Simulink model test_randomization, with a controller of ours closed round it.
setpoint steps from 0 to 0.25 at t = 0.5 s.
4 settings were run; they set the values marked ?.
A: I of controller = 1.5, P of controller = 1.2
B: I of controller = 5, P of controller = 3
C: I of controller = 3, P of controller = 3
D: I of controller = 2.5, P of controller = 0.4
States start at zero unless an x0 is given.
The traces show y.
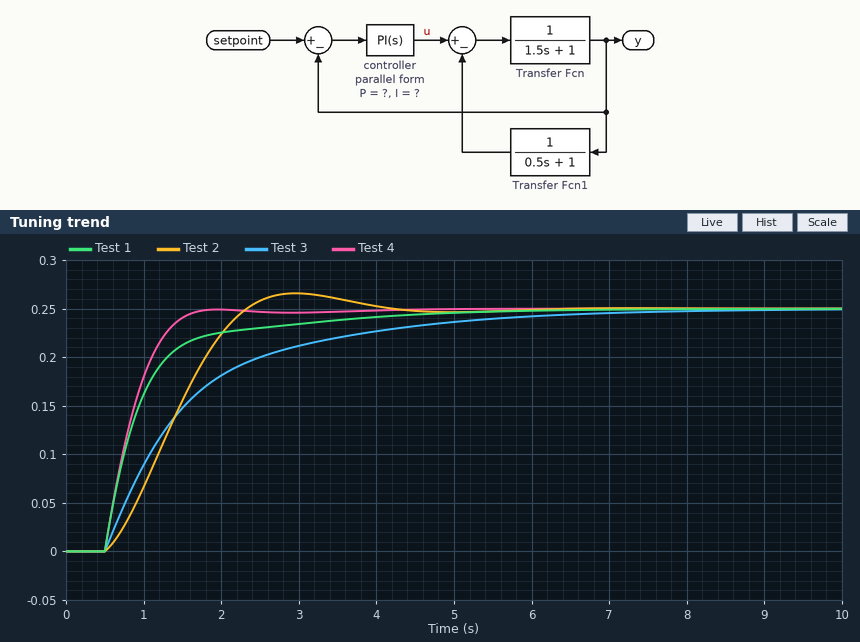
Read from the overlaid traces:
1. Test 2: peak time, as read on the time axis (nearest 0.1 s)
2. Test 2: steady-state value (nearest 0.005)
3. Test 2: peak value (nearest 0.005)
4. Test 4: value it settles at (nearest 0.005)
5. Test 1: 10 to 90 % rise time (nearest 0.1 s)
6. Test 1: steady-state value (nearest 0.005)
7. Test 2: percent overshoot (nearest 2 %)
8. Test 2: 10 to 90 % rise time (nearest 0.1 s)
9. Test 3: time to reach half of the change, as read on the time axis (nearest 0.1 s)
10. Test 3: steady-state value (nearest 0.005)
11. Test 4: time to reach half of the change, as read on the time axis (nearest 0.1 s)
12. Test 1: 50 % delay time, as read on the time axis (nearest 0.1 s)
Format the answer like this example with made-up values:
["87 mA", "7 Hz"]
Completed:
["3.0 s", "0.250", "0.265", "0.250", "1.4 s", "0.250", "6 %", "1.3 s", "1.3 s", "0.250", "0.8 s", "0.8 s"]
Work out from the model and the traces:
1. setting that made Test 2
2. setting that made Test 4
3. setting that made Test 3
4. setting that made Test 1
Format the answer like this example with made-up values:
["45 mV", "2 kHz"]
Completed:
["D", "B", "A", "C"]
